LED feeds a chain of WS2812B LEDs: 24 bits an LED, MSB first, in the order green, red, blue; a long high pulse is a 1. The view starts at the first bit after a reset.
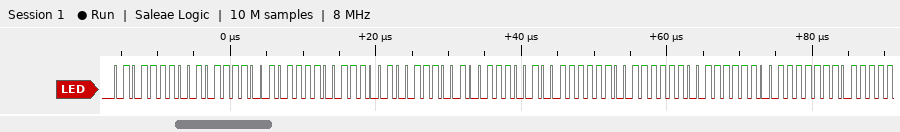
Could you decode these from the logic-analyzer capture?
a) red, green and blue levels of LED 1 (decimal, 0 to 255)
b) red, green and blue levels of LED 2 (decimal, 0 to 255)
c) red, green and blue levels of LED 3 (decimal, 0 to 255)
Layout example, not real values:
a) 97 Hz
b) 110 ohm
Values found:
a) 94, 94, 94
b) 114, 114, 114
c) 126, 126, 126
